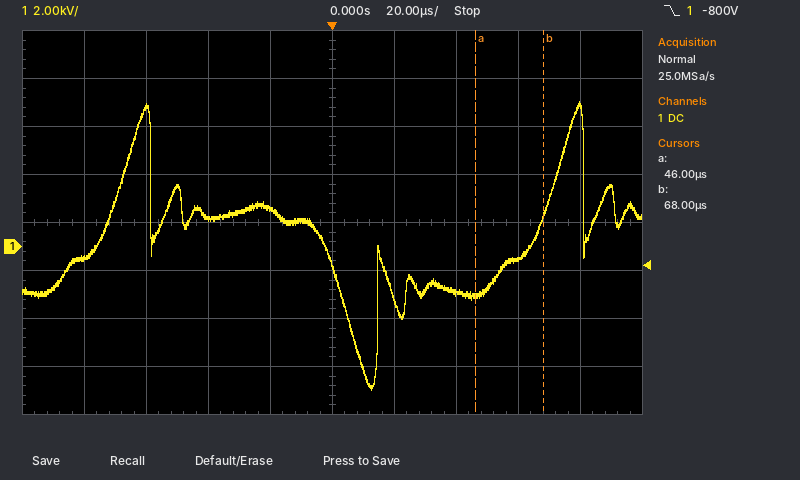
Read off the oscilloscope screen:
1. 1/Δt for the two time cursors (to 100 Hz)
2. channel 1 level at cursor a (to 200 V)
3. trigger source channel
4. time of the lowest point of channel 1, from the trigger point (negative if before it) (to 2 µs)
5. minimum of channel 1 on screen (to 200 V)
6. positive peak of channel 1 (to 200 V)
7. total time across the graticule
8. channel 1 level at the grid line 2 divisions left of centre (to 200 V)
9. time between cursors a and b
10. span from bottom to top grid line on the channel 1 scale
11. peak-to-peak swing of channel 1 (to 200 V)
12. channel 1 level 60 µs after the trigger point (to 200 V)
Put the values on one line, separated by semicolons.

45.5 kHz; -2.0 kV; channel 1; +12 µs; -6.0 kV; 6.0 kV; 200 µs; 1.2 kV; 22 µs; 16 kV; 12.0 kV; -600 V
